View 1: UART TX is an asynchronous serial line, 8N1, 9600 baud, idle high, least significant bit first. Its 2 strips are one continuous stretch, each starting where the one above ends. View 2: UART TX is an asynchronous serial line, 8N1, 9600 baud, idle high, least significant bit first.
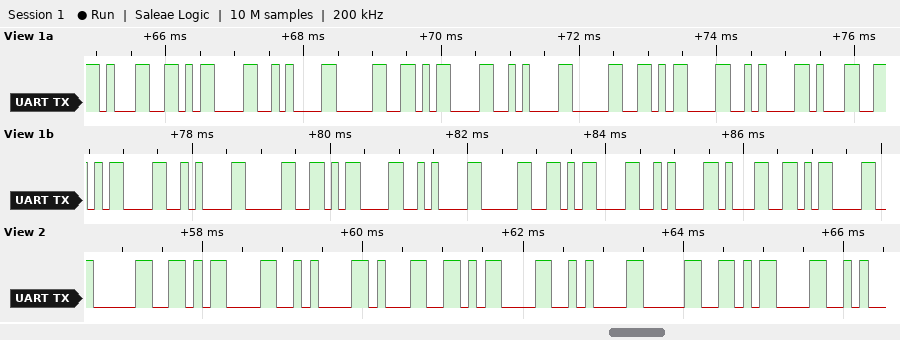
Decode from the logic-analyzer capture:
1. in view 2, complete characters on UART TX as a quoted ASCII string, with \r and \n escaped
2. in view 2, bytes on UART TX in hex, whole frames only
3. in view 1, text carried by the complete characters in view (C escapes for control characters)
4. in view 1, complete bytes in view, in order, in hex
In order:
"0\r\n1\r\n0\r"
0x30 0x0D 0x0A 0x31 0x0D 0x0A 0x30 0x0D
"1\r\n0\r\n0\r\n1\r\n0\r\n0\r\n1\r"
0x31 0x0D 0x0A 0x30 0x0D 0x0A 0x30 0x0D 0x0A 0x31 0x0D 0x0A 0x30 0x0D 0x0A 0x30 0x0D 0x0A 0x31 0x0D
